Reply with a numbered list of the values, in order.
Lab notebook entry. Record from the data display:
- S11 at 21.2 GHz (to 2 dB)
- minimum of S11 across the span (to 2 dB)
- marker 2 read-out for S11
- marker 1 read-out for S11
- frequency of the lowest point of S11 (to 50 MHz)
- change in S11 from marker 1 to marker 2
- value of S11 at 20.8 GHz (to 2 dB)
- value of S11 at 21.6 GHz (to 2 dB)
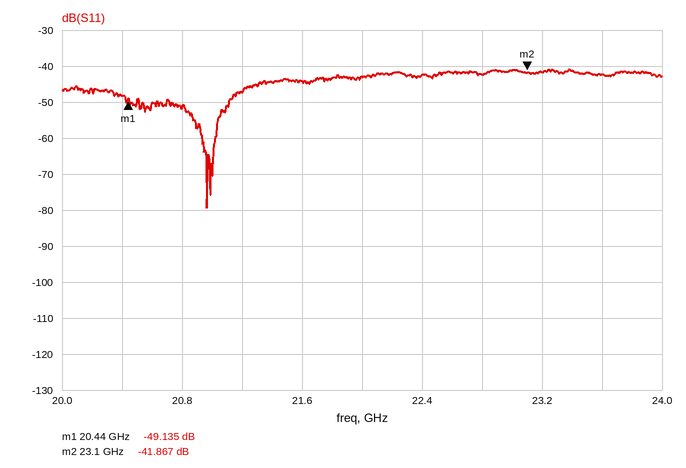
1. -48 dB
2. -80 dB
3. -41.867 dB
4. -49.135 dB
5. 20.95 GHz
6. 7.268 dB
7. -52 dB
8. -44 dB
